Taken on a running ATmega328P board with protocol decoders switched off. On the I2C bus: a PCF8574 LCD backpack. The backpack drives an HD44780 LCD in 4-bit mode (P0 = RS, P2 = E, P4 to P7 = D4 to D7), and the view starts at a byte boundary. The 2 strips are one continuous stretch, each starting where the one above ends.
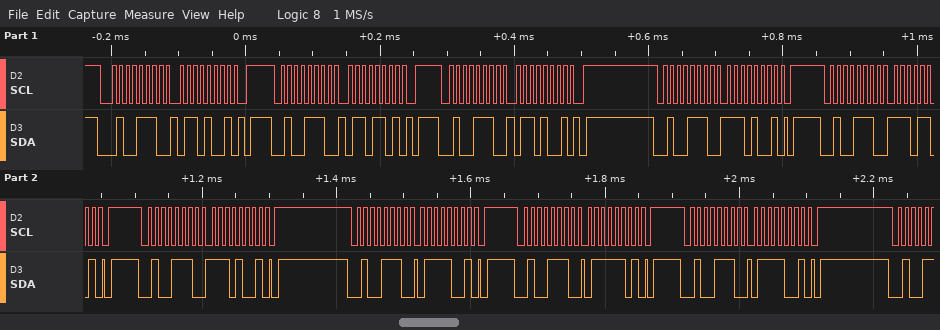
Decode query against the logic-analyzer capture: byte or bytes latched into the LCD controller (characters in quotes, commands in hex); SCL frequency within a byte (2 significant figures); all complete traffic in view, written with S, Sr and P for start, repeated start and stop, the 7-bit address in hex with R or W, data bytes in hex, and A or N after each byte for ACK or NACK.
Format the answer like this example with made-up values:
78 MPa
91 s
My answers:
'n'
100 kHz
S 27W A 69 A P S 27W A 6D A P S 27W A 69 A P S 27W A E9 A P S 27W A ED A P S 27W A E9 A P S 27W A 79 A P S 27W A 7D A P S 27W A 79 A P
